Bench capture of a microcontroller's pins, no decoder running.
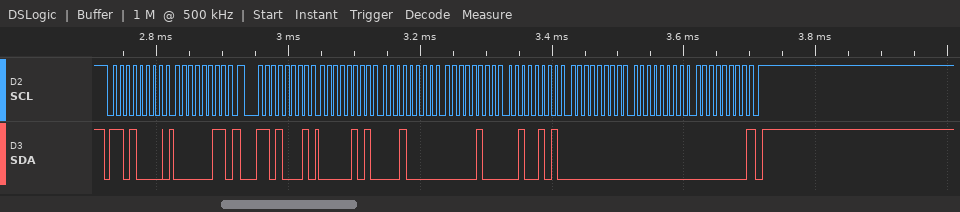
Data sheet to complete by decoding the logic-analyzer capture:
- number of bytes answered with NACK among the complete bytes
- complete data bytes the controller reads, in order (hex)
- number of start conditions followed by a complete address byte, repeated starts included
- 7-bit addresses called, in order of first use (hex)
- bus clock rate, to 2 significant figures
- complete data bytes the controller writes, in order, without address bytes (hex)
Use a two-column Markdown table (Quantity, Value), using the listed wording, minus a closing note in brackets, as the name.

| Quantity | Value |
|---|---|
| number of bytes answered with NACK among the complete bytes | 1 |
| complete data bytes the controller reads, in order | 05 10 04 25 00 00 00 |
| number of start conditions followed by a complete address byte, repeated starts included | 2 |
| 7-bit addresses called, in order of first use | 0x68 |
| bus clock rate, to 2 significant figures | 100 kHz |
| complete data bytes the controller writes, in order, without address bytes | 03 |
